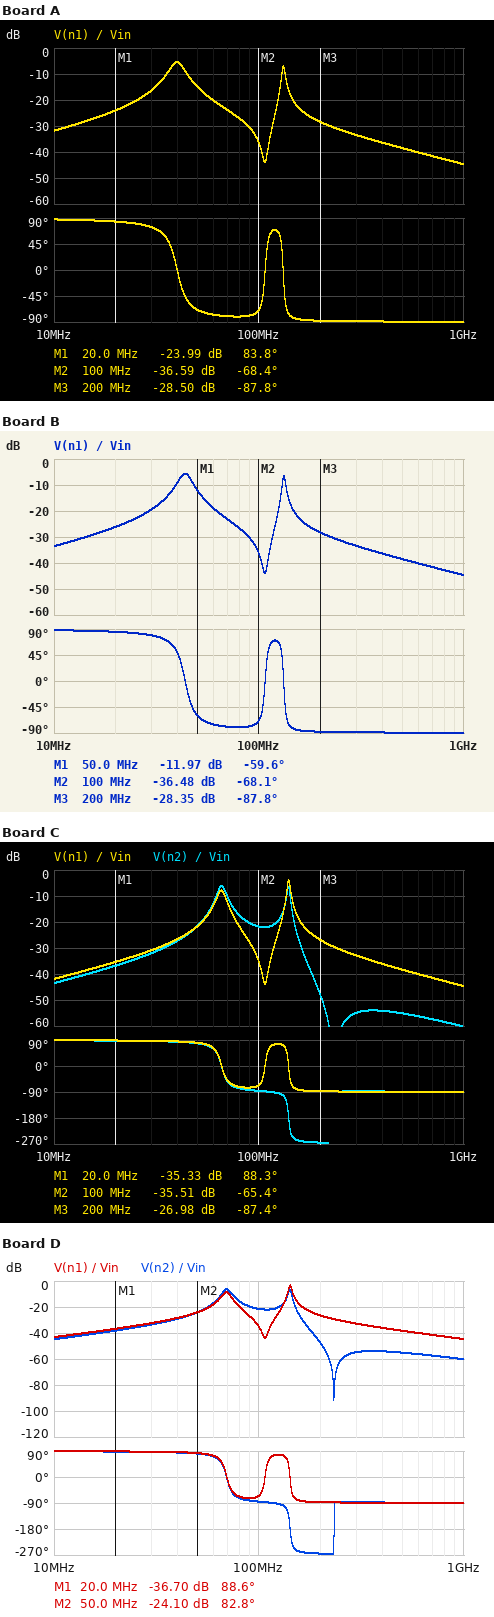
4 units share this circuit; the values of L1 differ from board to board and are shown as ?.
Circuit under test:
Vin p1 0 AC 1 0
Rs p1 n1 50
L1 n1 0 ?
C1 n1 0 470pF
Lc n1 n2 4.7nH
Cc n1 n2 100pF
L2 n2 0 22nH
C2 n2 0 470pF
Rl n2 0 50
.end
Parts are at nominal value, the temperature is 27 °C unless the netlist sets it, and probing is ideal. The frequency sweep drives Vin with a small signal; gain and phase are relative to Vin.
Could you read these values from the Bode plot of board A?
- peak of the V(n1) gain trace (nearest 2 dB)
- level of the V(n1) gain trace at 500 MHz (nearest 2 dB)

-6 dB
-38 dB
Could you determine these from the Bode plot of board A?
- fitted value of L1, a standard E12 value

68 nH
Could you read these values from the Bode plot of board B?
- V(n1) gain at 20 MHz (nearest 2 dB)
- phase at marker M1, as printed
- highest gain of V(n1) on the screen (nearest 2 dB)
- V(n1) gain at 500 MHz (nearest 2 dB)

-26 dB
-59.6 deg
-6 dB
-38 dB
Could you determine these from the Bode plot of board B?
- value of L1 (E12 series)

39 nH
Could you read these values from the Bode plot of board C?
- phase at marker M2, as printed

-65.4 deg
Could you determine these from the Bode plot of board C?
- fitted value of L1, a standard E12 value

8.2 nH
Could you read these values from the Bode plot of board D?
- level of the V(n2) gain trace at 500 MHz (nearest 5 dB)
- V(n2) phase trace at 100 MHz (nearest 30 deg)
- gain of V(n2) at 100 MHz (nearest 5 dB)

-55 dB
-90 deg
-20 dB
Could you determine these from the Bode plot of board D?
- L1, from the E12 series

6.8 nH
